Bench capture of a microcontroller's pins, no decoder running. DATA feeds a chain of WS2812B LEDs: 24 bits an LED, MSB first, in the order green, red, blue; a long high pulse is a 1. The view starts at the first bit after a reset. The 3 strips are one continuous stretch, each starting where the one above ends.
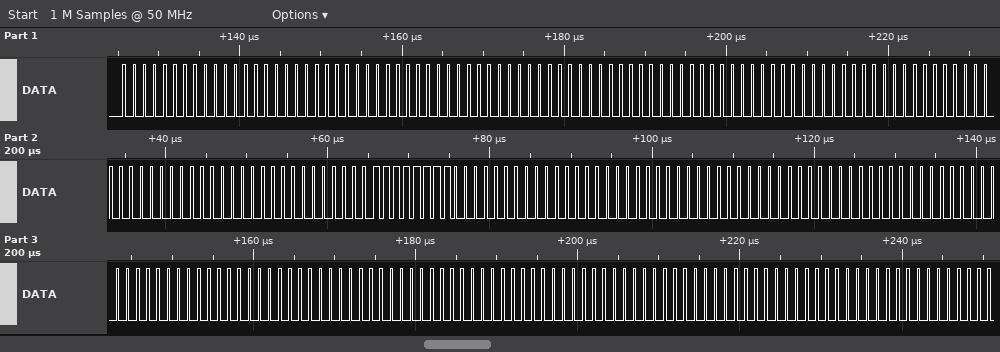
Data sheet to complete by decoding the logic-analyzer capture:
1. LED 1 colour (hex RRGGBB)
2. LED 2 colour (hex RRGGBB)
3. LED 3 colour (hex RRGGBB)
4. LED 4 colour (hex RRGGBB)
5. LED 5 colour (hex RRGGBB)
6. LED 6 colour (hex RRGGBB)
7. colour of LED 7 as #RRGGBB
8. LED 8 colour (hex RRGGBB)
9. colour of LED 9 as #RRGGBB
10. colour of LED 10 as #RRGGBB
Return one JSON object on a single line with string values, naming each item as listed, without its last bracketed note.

{"LED 1 colour": "#000000", "LED 2 colour": "#000000", "LED 3 colour": "#000000", "LED 4 colour": "#000000", "LED 5 colour": "#0000FF", "LED 6 colour": "#000000", "colour of LED 7 as #RRGGBB": "#000000", "LED 8 colour": "#000000", "colour of LED 9 as #RRGGBB": "#000000", "colour of LED 10 as #RRGGBB": "#000000"}
